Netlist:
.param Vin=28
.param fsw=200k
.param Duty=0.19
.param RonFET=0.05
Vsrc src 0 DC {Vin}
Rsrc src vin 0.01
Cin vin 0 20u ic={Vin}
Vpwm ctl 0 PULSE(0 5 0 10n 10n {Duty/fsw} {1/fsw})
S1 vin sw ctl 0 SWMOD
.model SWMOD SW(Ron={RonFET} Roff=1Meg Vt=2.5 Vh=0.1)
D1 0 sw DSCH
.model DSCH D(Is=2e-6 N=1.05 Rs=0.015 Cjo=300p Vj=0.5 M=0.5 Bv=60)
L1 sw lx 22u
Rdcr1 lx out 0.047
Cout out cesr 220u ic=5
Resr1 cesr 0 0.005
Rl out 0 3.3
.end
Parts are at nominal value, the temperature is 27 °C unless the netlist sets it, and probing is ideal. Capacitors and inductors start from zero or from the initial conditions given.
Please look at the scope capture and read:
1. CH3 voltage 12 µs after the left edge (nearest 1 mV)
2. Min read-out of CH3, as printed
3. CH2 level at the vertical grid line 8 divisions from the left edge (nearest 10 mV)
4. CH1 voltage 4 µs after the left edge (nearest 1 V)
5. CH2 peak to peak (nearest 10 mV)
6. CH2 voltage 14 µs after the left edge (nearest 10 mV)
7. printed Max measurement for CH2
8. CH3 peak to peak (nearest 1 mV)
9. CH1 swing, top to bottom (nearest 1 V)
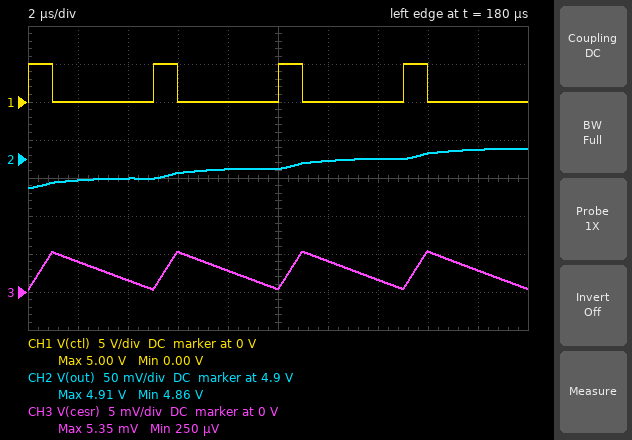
4 mV
250 µV
4.91 V
0 V
50 mV
4.90 V
4.91 V
5 mV
5 V
